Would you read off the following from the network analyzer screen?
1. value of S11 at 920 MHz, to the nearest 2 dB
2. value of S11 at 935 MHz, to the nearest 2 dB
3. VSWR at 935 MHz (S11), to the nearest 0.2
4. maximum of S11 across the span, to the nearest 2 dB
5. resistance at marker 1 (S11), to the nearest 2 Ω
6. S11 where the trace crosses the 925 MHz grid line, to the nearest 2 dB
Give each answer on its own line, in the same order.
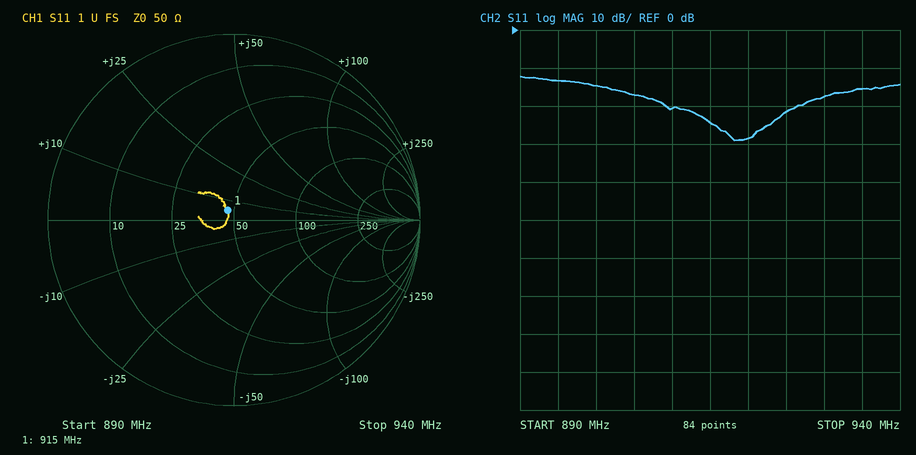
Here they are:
-28 dB
-16 dB
1.4
-12 dB
46 Ω
-22 dB
